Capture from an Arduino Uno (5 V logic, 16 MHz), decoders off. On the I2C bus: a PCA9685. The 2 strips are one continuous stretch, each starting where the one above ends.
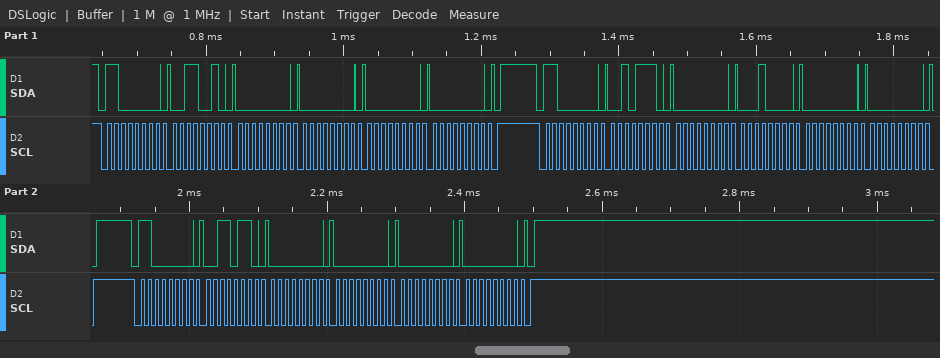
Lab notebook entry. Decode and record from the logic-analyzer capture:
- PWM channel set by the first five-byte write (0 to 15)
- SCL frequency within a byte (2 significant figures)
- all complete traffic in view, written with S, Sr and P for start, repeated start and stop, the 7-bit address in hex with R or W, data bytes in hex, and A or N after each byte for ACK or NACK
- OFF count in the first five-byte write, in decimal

11
100 kHz
S 60W A 32 A 00 A 00 A 00 A 00 A P S 60W A 2E A 00 A 10 A 00 A 00 A P S 60W A 36 A 00 A 00 A 00 A 00 A P
0
